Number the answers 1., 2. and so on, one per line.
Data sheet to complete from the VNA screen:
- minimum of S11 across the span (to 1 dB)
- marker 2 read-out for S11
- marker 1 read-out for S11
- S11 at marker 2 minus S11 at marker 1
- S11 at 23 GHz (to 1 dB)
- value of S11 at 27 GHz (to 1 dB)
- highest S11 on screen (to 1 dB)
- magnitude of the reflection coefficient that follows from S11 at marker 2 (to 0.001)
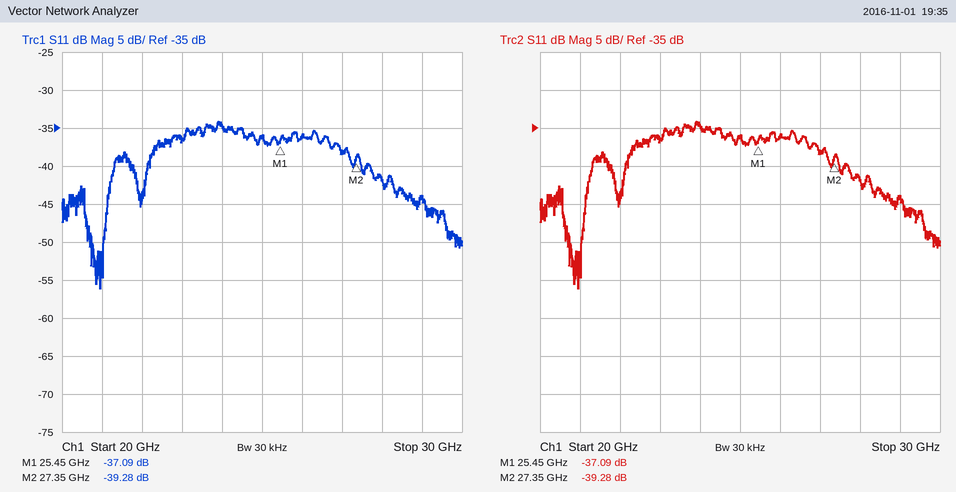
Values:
1. -56 dB
2. -39.28 dB
3. -37.09 dB
4. -2.19 dB
5. -36 dB
6. -38 dB
7. -34 dB
8. 0.011
